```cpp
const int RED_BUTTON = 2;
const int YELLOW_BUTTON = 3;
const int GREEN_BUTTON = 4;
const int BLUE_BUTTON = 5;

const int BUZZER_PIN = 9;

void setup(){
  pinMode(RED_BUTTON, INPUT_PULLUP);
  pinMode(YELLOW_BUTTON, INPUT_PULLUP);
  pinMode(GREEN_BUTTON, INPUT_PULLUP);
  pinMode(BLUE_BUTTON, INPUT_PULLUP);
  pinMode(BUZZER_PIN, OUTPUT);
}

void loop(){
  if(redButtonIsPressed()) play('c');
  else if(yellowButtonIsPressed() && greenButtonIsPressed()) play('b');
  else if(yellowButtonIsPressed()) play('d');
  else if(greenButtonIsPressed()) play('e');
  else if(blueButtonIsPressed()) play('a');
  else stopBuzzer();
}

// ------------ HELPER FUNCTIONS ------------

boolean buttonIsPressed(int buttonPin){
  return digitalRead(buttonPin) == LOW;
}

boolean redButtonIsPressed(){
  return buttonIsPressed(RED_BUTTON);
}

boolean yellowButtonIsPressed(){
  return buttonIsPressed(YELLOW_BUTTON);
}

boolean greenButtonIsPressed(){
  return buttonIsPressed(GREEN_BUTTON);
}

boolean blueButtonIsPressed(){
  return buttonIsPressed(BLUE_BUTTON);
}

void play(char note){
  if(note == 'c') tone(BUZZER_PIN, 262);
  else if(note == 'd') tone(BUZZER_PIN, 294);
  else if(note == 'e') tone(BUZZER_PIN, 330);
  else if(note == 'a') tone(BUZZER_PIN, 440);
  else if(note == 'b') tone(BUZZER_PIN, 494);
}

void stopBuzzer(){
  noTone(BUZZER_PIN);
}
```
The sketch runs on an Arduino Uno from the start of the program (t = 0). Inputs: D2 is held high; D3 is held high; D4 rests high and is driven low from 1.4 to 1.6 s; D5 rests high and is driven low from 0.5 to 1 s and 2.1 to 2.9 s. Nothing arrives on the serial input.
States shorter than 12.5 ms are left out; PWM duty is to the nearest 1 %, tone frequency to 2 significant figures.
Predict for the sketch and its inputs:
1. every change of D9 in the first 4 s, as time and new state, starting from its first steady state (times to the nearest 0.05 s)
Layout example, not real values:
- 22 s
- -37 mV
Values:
- 0 s low; 0.5 s tone 440 Hz; 1 s low; 1.4 s tone 330 Hz; 1.6 s low; 2.1 s tone 440 Hz; 2.9 s low
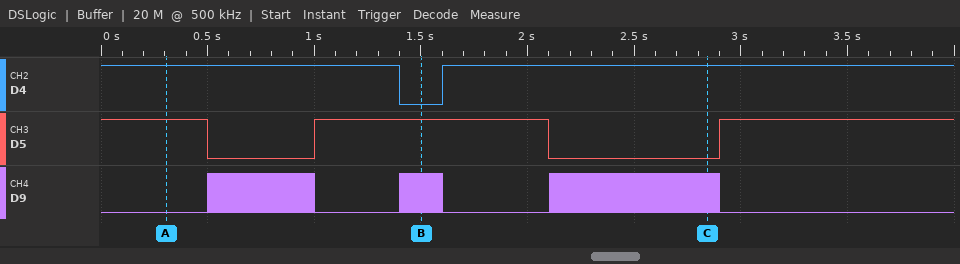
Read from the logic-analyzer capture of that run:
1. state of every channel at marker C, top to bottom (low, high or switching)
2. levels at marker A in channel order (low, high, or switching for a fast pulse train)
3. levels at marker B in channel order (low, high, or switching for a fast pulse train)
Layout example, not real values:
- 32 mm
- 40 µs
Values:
- D4 high, D5 low, D9 switching
- D4 high, D5 high, D9 low
- D4 low, D5 high, D9 switching
